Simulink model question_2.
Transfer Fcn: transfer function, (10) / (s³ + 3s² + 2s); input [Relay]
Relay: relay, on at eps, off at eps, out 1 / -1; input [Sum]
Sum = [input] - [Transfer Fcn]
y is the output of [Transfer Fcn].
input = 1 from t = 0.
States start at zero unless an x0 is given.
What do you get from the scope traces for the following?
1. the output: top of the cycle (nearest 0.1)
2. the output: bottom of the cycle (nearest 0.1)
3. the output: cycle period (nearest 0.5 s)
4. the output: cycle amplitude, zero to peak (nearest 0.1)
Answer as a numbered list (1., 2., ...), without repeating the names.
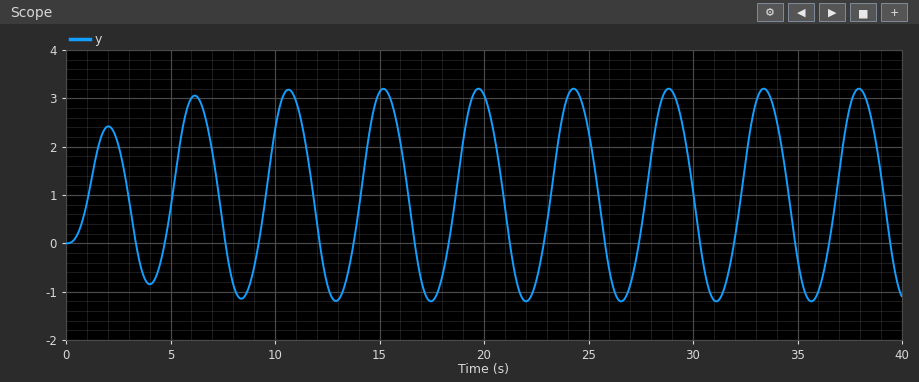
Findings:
1. 3.2
2. -1.2
3. 4.5 s
4. 2.2
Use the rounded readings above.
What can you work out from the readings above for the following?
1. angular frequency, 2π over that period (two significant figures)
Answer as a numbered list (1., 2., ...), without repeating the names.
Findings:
1. 1.4 rad/s
